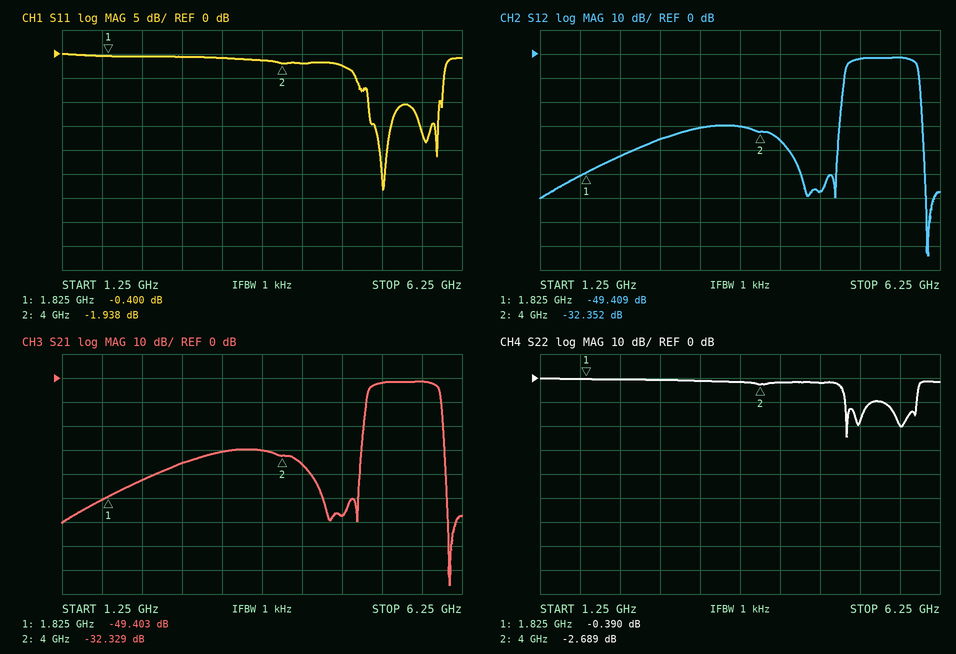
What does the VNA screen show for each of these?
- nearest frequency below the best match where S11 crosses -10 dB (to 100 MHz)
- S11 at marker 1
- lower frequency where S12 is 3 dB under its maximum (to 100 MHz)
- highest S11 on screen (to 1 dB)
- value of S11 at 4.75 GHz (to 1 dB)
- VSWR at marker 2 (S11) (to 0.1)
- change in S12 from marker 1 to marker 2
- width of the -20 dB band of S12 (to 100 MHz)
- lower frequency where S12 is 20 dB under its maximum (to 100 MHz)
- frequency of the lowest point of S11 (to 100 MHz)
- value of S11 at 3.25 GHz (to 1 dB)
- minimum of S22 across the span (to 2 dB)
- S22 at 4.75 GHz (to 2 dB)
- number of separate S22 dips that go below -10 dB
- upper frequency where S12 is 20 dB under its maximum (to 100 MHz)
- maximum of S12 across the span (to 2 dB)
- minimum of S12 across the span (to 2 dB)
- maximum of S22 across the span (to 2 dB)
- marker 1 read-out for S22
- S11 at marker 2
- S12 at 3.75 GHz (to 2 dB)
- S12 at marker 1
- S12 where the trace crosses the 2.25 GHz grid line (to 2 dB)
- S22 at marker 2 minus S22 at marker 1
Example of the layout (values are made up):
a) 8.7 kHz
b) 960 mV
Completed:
a) 5.1 GHz
b) -0.400 dB
c) 5.1 GHz
d) 0 dB
e) -2 dB
f) 9.0
g) 17.057 dB
h) 1.0 GHz
i) 5.0 GHz
j) 5.3 GHz
k) -1 dB
l) -24 dB
m) -2 dB
n) 3
o) 6.0 GHz
p) -2 dB
q) -84 dB
r) 0 dB
s) -0.390 dB
t) -1.938 dB
u) -30 dB
v) -49.409 dB
w) -42 dB
x) -2.299 dB
